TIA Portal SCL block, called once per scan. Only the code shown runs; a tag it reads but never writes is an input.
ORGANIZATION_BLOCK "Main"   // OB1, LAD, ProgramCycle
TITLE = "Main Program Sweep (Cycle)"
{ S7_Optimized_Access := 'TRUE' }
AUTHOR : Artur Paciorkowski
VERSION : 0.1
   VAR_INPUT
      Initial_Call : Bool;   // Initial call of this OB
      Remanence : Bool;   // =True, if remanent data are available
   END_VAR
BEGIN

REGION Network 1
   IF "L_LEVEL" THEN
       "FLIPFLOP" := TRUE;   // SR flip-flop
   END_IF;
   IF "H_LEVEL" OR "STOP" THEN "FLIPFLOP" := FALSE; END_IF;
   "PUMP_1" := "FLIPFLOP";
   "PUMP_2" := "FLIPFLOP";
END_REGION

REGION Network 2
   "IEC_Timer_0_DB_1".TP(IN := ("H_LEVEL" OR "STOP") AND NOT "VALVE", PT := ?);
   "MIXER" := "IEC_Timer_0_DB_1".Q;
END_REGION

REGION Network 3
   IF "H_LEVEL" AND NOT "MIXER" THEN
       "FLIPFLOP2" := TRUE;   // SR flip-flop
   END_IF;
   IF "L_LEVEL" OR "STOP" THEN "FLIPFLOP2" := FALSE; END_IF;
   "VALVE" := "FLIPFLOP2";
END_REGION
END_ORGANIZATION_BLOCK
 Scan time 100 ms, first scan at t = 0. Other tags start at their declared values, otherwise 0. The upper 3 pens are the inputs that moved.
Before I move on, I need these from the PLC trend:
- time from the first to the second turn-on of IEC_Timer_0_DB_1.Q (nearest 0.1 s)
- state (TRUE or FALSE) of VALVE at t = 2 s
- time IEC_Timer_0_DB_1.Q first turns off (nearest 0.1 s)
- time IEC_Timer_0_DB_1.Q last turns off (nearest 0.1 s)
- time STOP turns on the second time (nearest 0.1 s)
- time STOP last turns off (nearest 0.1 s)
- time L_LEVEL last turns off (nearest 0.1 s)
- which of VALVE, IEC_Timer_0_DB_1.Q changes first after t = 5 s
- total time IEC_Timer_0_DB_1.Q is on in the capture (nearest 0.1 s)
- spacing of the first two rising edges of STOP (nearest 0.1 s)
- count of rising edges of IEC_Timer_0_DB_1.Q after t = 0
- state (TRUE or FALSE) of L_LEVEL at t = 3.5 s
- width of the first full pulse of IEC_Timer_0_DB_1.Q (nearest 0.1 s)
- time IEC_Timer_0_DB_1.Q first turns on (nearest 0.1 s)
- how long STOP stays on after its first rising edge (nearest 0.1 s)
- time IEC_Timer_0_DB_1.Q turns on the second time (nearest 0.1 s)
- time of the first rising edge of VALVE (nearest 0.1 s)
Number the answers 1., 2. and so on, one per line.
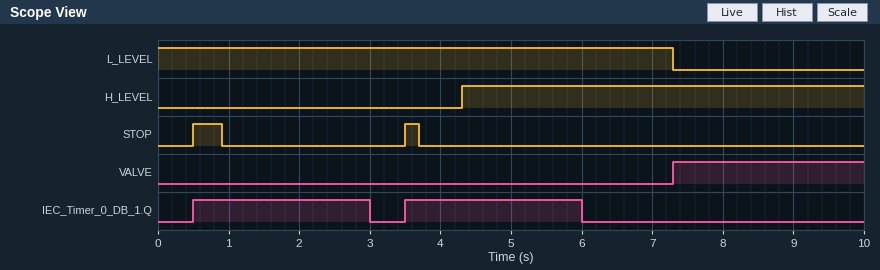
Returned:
1. 3.0 s
2. FALSE
3. 3.0 s
4. 6.0 s
5. 3.5 s
6. 3.7 s
7. 7.3 s
8. IEC_Timer_0_DB_1.Q
9. 5.0 s
10. 3.0 s
11. 2
12. TRUE
13. 2.5 s
14. 0.5 s
15. 0.4 s
16. 3.5 s
17. 7.3 s
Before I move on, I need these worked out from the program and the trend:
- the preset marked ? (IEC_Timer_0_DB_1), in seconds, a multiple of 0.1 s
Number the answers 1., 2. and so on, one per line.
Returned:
1. 2.5 s
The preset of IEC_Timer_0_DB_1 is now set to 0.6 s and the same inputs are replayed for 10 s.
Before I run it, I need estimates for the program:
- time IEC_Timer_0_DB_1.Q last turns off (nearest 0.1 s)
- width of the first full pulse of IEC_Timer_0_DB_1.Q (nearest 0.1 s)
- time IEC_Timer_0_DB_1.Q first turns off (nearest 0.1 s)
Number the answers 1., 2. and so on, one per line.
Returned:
1. 4.9 s
2. 0.6 s
3. 1.1 s
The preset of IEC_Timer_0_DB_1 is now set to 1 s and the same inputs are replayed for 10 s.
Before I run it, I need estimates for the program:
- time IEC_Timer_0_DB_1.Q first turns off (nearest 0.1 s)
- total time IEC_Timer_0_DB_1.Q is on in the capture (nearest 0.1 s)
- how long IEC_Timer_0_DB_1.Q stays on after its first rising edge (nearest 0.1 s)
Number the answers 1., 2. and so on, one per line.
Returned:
1. 1.5 s
2. 2.0 s
3. 1.0 s
